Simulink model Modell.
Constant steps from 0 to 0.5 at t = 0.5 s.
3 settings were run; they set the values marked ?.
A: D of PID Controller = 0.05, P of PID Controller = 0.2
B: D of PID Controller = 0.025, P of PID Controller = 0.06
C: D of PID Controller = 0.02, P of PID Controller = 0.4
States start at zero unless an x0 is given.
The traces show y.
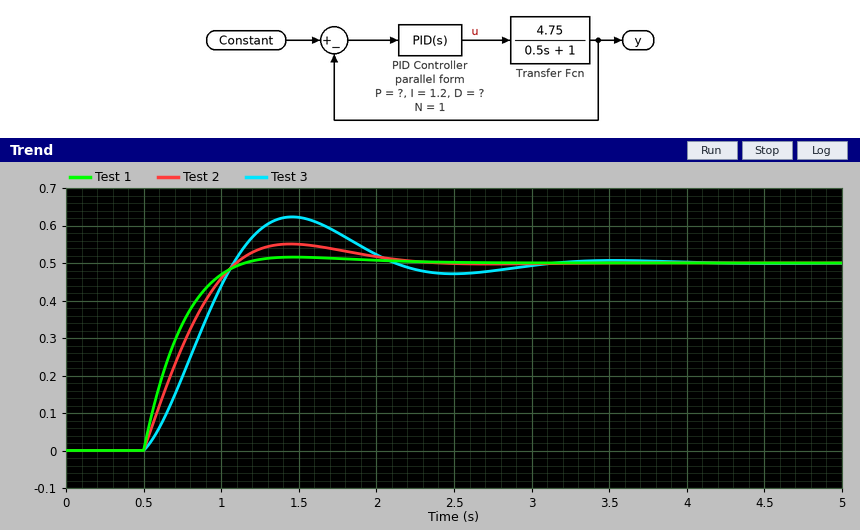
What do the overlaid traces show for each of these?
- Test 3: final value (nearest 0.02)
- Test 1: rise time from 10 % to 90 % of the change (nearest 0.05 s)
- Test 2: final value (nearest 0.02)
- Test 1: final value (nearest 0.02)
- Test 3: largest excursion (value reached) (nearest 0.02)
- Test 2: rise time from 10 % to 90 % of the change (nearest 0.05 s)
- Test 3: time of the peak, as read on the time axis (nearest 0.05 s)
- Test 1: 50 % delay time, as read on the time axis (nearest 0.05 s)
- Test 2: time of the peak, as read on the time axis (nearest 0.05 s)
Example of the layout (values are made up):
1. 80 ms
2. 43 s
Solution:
1. 0.50
2. 0.40 s
3. 0.50
4. 0.50
5. 0.62
6. 0.45 s
7. 1.45 s
8. 0.65 s
9. 1.45 s
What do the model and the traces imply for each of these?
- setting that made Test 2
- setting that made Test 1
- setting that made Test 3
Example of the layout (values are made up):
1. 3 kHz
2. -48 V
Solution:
1. A
2. C
3. B
